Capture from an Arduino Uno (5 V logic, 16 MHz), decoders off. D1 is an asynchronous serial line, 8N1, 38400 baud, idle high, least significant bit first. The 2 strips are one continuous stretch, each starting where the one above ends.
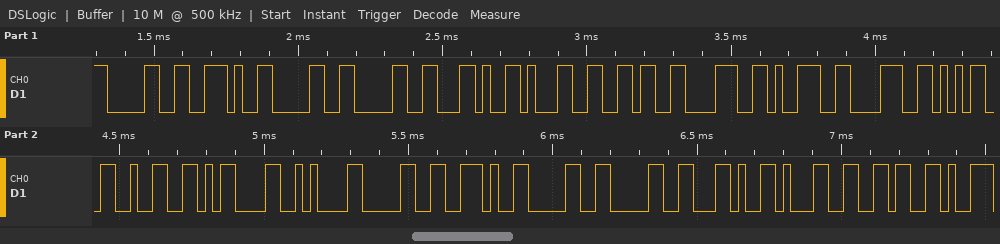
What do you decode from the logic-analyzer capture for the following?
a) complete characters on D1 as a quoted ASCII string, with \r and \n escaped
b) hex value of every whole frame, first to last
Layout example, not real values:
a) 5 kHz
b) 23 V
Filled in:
a) "0.00,1689852\r\n0.00,16"
b) 30 2E 30 30 2C 31 36 38 39 38 35 32 0D 0A 30 2E 30 30 2C 31 36
